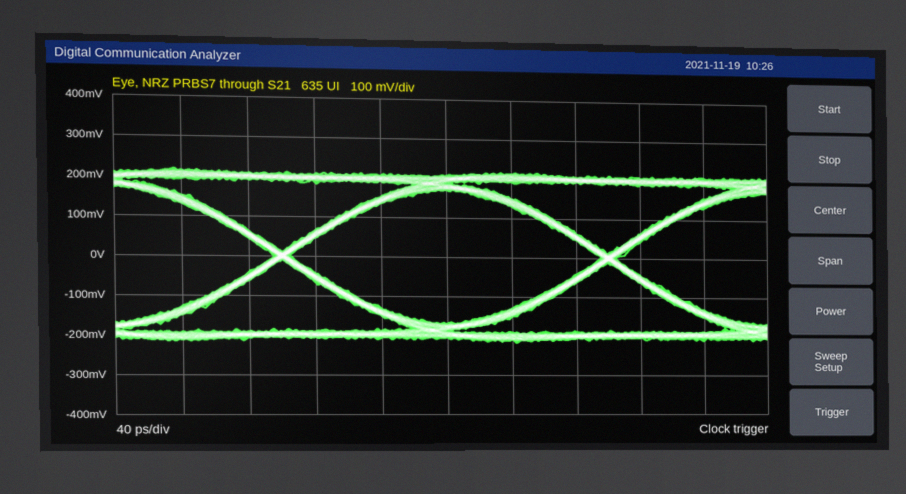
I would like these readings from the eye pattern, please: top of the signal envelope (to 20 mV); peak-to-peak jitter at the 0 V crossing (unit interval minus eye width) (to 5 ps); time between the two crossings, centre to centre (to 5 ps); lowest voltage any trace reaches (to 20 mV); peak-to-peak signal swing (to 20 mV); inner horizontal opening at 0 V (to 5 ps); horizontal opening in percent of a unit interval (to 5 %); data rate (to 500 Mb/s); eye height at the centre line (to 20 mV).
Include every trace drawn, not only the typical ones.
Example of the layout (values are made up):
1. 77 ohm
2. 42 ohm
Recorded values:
1. 220 mV
2. 10 ps
3. 200 ps
4. -220 mV
5. 440 mV
6. 190 ps
7. 95 %
8. 5.0 Gb/s
9. 340 mV
